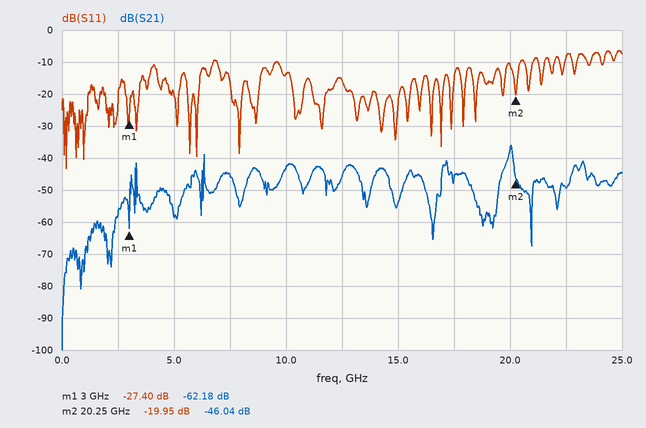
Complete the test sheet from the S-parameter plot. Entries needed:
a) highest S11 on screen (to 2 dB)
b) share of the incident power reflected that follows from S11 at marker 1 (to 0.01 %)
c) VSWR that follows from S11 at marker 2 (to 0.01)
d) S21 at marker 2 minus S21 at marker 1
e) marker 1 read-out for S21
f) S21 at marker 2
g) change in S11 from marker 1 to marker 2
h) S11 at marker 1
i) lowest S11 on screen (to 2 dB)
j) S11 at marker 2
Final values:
-6 dB
0.18 %
1.22
16.14 dB
-62.18 dB
-46.04 dB
7.45 dB
-27.40 dB
-44 dB
-19.95 dB
